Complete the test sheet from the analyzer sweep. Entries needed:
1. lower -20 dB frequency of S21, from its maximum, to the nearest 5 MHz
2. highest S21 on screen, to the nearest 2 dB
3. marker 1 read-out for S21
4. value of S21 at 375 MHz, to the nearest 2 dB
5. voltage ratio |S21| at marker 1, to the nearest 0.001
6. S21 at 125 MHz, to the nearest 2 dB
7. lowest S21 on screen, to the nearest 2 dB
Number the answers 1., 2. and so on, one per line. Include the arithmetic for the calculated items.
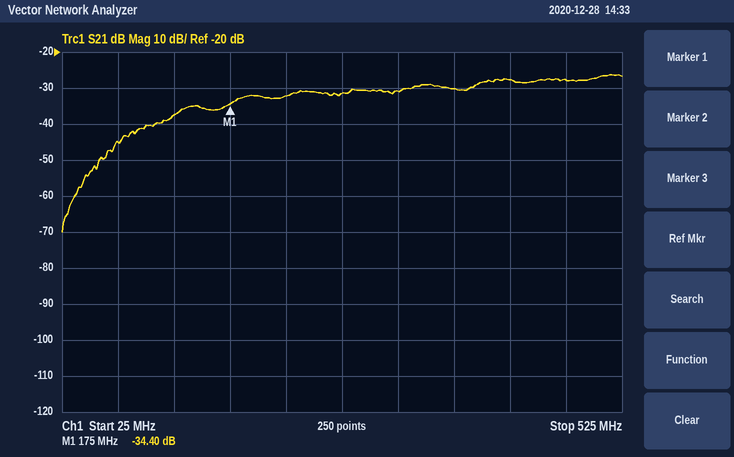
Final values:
1. 70 MHz
2. -26 dB
3. -34.40 dB
4. -30 dB
5. 10^(-34.4/20) ≈ 0.019
6. -38 dB
7. -70 dB
